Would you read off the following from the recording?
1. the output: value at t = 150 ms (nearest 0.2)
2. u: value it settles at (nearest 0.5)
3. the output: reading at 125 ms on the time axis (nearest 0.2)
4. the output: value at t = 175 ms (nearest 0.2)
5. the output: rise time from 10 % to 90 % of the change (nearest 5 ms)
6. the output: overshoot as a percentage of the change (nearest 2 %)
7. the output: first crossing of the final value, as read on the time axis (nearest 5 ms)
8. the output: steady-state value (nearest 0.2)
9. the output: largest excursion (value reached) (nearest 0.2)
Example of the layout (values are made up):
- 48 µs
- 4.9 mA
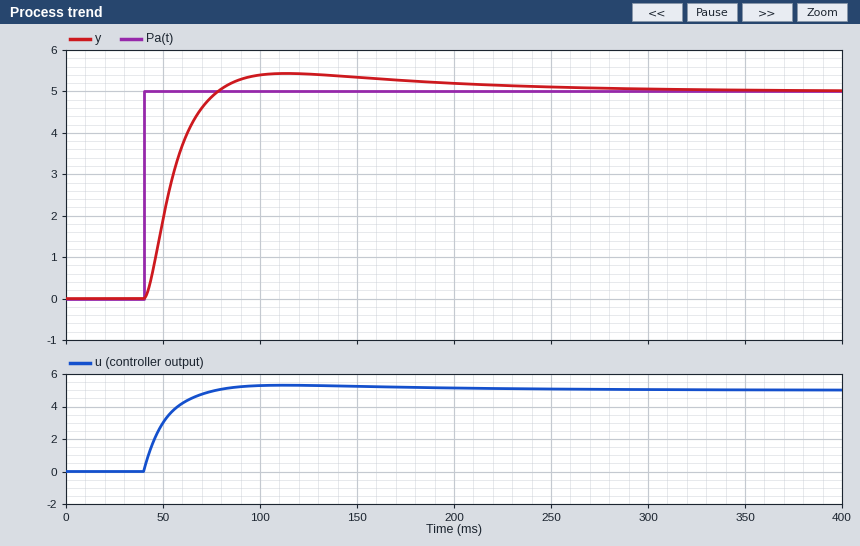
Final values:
- 5.4
- 5.0
- 5.4
- 5.2
- 25 ms
- 8 %
- 80 ms
- 5.0
- 5.4
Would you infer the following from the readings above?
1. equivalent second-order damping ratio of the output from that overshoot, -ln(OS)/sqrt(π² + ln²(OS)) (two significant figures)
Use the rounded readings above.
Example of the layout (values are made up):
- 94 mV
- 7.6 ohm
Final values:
- 0.63
